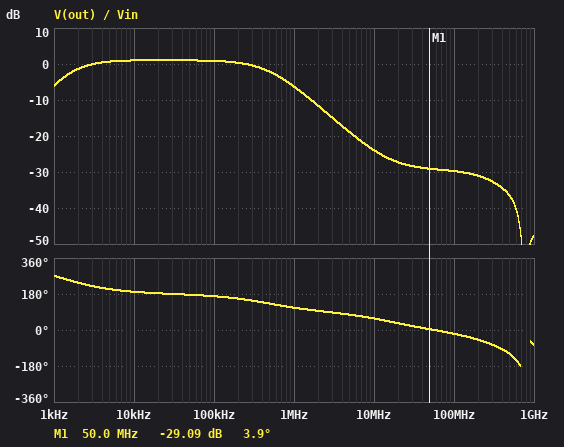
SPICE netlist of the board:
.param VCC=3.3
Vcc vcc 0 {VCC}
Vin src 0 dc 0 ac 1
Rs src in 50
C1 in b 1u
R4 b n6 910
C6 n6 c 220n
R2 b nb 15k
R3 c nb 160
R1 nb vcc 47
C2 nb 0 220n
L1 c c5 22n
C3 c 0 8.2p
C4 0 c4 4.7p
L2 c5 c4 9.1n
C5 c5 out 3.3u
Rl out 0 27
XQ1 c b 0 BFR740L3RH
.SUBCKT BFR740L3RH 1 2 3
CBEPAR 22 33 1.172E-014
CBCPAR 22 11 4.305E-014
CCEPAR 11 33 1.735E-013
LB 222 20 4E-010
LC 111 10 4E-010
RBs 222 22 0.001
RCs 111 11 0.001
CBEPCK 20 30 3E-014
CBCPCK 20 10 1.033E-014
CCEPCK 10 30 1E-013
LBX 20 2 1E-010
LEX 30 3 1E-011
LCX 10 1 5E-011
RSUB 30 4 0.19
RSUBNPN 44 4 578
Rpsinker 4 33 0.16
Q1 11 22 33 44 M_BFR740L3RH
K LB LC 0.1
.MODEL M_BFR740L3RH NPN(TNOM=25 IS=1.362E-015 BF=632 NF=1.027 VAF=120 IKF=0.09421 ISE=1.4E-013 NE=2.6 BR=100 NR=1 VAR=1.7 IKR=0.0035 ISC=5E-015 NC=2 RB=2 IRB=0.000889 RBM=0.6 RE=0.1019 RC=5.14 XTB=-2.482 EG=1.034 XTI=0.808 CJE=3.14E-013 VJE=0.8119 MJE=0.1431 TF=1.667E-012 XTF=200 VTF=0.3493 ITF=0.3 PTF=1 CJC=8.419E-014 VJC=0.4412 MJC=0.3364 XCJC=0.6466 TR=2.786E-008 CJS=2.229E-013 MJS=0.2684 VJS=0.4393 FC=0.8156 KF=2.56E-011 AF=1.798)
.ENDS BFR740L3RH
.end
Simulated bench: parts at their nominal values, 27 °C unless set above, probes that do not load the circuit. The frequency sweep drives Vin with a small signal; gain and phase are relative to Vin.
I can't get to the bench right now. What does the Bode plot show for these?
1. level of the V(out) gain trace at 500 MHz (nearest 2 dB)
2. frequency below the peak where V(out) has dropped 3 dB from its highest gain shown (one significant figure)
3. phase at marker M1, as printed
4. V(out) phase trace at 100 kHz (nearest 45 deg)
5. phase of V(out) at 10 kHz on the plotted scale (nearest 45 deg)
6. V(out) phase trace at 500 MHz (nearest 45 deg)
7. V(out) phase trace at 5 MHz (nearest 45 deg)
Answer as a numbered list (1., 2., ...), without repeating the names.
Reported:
1. -36 dB
2. 2 kHz
3. 3.9 deg
4. 180 deg
5. 180 deg
6. -135 deg
7. 90 deg
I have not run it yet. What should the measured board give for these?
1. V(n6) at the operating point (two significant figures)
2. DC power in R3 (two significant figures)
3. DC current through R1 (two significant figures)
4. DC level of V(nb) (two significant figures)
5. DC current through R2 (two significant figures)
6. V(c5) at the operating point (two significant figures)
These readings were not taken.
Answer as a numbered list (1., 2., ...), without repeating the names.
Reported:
1. 830 mV
2. 36 mW
3. 15 mA
4. 2.6 V
5. 120 µA
6. 180 mV
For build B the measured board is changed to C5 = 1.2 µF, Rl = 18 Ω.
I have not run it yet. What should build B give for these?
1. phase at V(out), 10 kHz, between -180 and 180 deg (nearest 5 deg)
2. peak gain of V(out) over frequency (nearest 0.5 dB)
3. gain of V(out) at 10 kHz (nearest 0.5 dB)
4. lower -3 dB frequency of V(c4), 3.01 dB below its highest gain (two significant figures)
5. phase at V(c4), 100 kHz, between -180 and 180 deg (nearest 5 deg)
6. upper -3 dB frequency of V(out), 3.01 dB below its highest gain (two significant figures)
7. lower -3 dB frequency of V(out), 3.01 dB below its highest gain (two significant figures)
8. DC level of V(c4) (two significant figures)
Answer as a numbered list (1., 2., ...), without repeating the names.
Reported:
1. -150 deg
2. 0 dB
3. -1.0 dB
4. 760 Hz
5. 165 deg
6. 500 kHz
7. 4.6 kHz
8. 180 mV
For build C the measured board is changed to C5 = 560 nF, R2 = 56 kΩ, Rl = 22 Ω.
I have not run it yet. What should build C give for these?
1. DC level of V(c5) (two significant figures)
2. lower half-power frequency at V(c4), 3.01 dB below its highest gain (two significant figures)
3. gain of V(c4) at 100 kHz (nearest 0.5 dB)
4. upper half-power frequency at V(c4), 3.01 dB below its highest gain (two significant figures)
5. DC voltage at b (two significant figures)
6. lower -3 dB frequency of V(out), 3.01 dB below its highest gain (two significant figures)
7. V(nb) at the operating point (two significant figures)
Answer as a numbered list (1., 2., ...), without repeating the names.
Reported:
1. 1.2 V
2. 1.2 kHz
3. 11.5 dB
4. 7.5 kHz
5. 810 mV
6. 3.9 kHz
7. 2.8 V
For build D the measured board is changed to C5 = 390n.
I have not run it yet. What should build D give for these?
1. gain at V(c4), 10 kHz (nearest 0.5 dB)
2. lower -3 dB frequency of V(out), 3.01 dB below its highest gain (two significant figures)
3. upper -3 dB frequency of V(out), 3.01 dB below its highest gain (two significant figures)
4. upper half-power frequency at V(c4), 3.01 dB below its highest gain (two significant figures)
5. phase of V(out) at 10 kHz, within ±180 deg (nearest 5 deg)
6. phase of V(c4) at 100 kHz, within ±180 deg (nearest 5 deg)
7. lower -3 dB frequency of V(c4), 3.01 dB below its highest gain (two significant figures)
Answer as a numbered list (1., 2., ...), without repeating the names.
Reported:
1. 3.0 dB
2. 10 kHz
3. 500 kHz
4. 170 kHz
5. -130 deg
6. 165 deg
7. 920 Hz
